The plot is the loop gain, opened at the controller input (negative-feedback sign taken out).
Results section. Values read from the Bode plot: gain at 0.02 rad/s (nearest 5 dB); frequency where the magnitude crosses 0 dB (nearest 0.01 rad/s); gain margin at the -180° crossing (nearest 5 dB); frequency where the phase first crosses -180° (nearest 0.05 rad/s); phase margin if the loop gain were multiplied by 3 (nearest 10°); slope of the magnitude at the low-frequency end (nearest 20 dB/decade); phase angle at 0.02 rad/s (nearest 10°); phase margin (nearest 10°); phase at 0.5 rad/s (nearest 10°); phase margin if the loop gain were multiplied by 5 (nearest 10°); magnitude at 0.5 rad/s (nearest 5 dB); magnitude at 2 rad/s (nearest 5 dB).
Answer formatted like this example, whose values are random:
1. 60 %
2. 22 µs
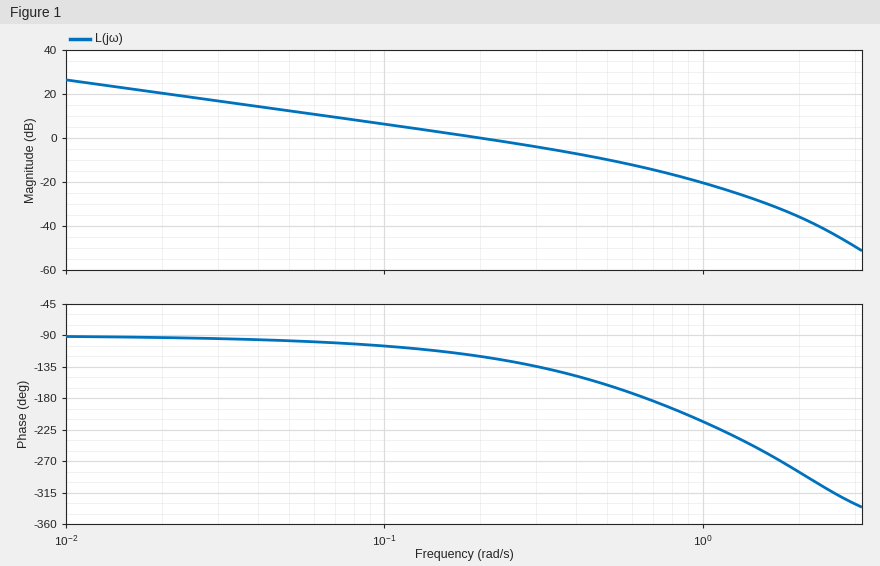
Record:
1. 20 dB
2. 0.20 rad/s
3. 15 dB
4. 0.65 rad/s
5. 20°
6. -20 dB/decade
7. -90°
8. 60°
9. -160°
10. 0°
11. -10 dB
12. -35 dB
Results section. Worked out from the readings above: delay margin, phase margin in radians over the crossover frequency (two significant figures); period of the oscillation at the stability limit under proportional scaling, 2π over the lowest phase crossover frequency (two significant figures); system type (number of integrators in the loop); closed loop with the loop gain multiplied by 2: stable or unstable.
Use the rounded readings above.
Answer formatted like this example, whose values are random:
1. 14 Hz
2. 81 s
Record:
1. 5.2 s
2. 9.7 s
3. 1
4. stable
